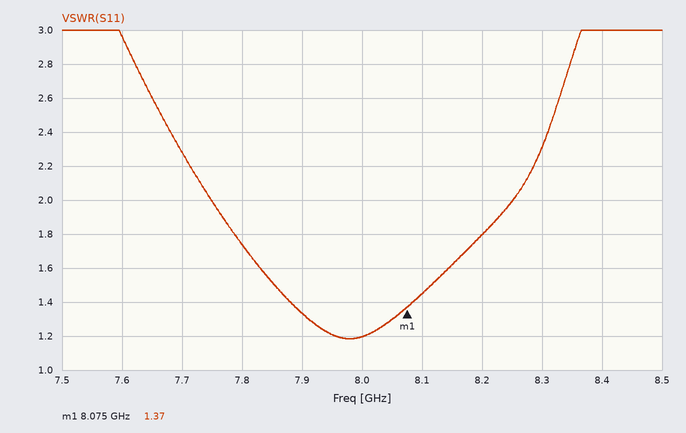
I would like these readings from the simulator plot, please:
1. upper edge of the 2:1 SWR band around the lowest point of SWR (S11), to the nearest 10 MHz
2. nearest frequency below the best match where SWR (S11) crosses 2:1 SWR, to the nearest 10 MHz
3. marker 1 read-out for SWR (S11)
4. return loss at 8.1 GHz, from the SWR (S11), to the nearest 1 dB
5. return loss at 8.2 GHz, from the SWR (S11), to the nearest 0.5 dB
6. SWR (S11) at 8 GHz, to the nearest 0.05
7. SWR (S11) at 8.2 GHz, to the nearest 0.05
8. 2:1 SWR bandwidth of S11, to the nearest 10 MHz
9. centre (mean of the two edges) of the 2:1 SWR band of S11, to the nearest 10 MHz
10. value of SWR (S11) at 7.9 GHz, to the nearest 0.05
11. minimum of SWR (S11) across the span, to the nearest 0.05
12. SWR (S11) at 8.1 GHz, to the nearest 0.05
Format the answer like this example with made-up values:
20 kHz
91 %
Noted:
8.25 GHz
7.75 GHz
1.37
15 dB
11.0 dB
1.20
1.80
500 MHz
8.00 GHz
1.35
1.20
1.45
